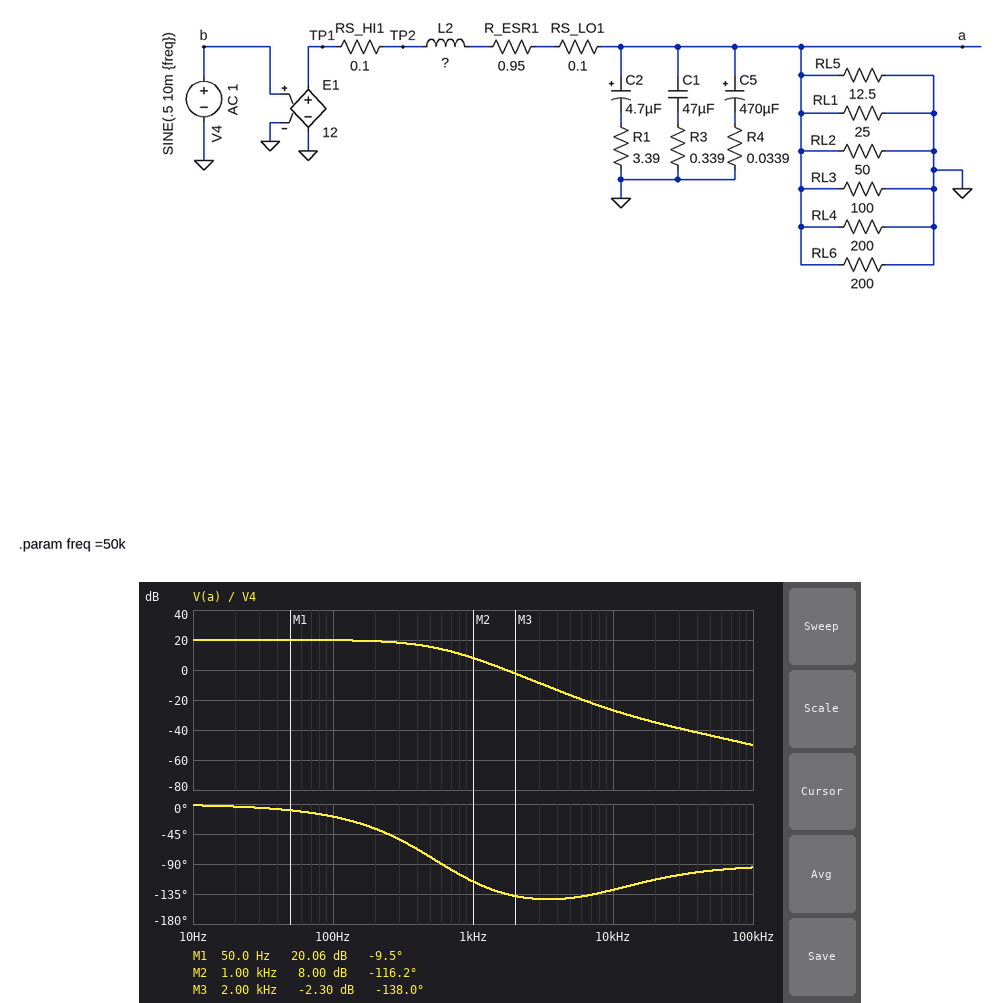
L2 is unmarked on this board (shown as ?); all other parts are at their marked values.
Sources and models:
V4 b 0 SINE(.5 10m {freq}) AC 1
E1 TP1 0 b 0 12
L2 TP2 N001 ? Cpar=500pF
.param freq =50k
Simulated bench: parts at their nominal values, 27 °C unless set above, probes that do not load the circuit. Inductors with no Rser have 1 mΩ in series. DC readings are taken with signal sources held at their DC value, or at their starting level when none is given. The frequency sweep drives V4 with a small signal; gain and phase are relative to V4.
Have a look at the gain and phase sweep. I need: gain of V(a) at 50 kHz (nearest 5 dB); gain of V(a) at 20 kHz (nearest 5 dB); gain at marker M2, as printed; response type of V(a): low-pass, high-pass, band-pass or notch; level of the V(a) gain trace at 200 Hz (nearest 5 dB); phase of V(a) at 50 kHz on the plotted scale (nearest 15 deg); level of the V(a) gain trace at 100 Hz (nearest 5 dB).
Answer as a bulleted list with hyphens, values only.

- -45 dB
- -35 dB
- 8.00 dB
- low-pass
- 20 dB
- -105 deg
- 20 dB
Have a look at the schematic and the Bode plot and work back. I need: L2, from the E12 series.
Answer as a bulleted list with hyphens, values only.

- 180 µH
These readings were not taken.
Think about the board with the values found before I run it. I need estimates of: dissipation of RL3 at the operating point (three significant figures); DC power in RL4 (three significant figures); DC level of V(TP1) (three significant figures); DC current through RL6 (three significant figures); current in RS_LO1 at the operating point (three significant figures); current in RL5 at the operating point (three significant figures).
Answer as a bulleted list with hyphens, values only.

- 257 mW
- 128 mW
- 6.00 V
- 25.3 mA
- 811 mA
- 405 mA
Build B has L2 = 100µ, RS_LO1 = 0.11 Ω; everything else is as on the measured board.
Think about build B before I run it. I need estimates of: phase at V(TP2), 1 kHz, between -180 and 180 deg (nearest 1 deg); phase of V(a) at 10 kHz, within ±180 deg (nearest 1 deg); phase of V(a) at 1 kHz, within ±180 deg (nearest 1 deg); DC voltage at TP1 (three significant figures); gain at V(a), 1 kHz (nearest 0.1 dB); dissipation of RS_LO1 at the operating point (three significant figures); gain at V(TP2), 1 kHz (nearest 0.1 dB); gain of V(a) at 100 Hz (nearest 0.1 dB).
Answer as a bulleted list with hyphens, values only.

- 1 deg
- -124 deg
- -97 deg
- 6.00 V
- 9.3 dB
- 72.1 mW
- 20.9 dB
- 19.8 dB
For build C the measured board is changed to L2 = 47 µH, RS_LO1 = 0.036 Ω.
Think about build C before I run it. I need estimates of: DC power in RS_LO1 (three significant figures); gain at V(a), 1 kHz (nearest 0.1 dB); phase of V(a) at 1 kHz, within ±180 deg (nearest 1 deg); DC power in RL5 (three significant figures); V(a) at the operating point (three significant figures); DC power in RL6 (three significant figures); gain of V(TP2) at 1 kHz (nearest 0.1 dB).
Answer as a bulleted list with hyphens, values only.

- 24.1 mW
- 10.2 dB
- -81 deg
- 2.09 W
- 5.11 V
- 131 mW
- 20.8 dB
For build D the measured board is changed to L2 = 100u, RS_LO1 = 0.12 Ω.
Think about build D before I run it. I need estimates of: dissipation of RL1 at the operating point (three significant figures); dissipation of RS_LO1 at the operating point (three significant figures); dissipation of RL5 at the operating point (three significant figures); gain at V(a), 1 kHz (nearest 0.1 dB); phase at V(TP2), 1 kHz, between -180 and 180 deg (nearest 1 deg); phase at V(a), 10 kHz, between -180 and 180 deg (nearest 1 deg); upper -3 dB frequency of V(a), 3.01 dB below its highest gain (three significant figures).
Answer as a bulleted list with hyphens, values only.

- 1.02 W
- 78.4 mW
- 2.04 W
- 9.3 dB
- 1 deg
- -124 deg
- 342 Hz
